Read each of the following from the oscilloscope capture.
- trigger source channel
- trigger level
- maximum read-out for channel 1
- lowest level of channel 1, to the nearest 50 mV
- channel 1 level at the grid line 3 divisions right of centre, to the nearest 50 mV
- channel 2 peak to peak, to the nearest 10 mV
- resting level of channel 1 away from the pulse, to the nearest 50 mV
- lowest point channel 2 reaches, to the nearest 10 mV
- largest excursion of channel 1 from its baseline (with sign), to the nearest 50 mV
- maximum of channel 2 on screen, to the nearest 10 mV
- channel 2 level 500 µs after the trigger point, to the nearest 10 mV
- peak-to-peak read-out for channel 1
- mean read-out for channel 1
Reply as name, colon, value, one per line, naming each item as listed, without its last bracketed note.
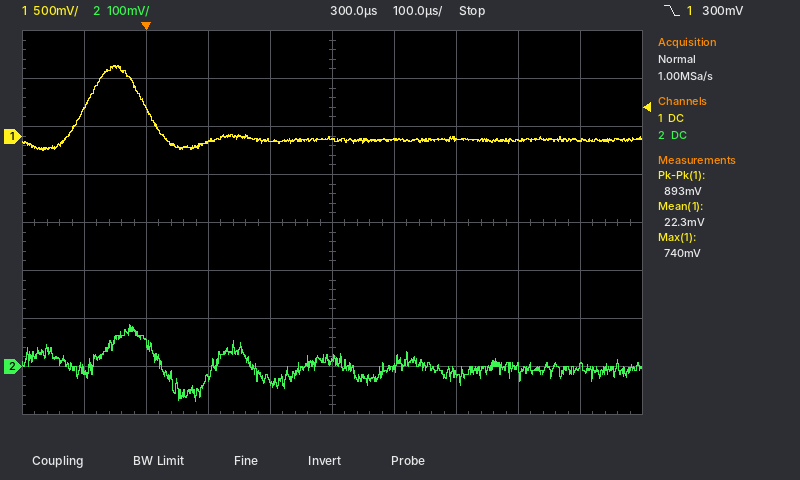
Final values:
trigger source channel: channel 1
trigger level: 300 mV
maximum read-out for channel 1: 740 mV
lowest level of channel 1, to the nearest 50 mV: -150 mV
channel 1 level at the grid line 3 divisions right of centre, to the nearest 50 mV: -50 mV
channel 2 peak to peak, to the nearest 10 mV: 160 mV
resting level of channel 1 away from the pulse, to the nearest 50 mV: -50 mV
lowest point channel 2 reaches, to the nearest 10 mV: -70 mV
largest excursion of channel 1 from its baseline (with sign), to the nearest 50 mV: +800 mV
maximum of channel 2 on screen, to the nearest 10 mV: 90 mV
channel 2 level 500 µs after the trigger point, to the nearest 10 mV: -10 mV
peak-to-peak read-out for channel 1: 893 mV
mean read-out for channel 1: 22.3 mV
